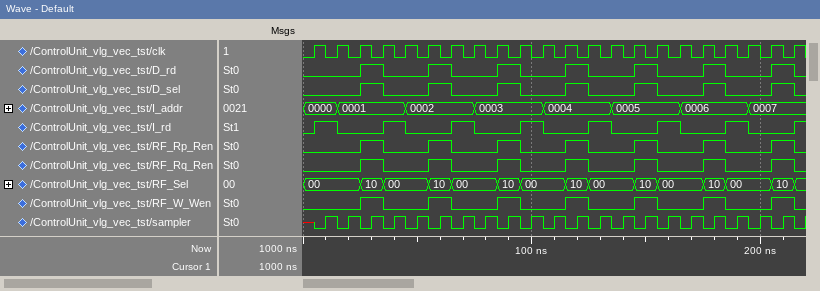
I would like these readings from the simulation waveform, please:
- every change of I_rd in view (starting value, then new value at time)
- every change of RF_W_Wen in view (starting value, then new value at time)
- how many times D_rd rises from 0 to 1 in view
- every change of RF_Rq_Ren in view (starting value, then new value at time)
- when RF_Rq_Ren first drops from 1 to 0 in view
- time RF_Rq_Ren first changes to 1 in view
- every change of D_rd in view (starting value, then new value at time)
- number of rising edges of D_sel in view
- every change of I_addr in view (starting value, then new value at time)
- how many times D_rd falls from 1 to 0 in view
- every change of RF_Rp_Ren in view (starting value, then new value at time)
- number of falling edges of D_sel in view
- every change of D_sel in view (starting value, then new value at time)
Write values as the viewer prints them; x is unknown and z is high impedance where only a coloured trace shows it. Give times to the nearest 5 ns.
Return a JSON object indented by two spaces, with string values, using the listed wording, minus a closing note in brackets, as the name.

{
  "every change of I_rd in view": "0, 1 at 5 ns, 0 at 15 ns, 1 at 35 ns, 0 at 45 ns, 1 at 65 ns, 0 at 75 ns, 1 at 95 ns, 0 at 105 ns, 1 at 125 ns, 0 at 135 ns, 1 at 155 ns, 0 at 165 ns, 1 at 185 ns, 0 at 195 ns, 1 at 215 ns",
  "every change of RF_W_Wen in view": "0, 1 at 25 ns, 0 at 35 ns, 1 at 55 ns, 0 at 65 ns, 1 at 85 ns, 0 at 95 ns, 1 at 115 ns, 0 at 125 ns, 1 at 145 ns, 0 at 155 ns, 1 at 175 ns, 0 at 185 ns, 1 at 205 ns, 0 at 215 ns",
  "how many times D_rd rises from 0 to 1 in view": "7",
  "every change of RF_Rq_Ren in view": "0, 1 at 25 ns, 0 at 35 ns, 1 at 55 ns, 0 at 65 ns, 1 at 85 ns, 0 at 95 ns, 1 at 115 ns, 0 at 125 ns, 1 at 145 ns, 0 at 155 ns, 1 at 175 ns, 0 at 185 ns, 1 at 205 ns, 0 at 215 ns",
  "when RF_Rq_Ren first drops from 1 to 0 in view": "35 ns",
  "time RF_Rq_Ren first changes to 1 in view": "25 ns",
  "every change of D_rd in view": "0, 1 at 25 ns, 0 at 35 ns, 1 at 55 ns, 0 at 65 ns, 1 at 85 ns, 0 at 95 ns, 1 at 115 ns, 0 at 125 ns, 1 at 145 ns, 0 at 155 ns, 1 at 175 ns, 0 at 185 ns, 1 at 205 ns, 0 at 215 ns",
  "number of rising edges of D_sel in view": "7",
  "every change of I_addr in view": "0000, 0001 at 15 ns, 0002 at 45 ns, 0003 at 75 ns, 0004 at 105 ns, 0005 at 135 ns, 0006 at 165 ns, 0007 at 195 ns",
  "how many times D_rd falls from 1 to 0 in view": "7",
  "every change of RF_Rp_Ren in view": "0, 1 at 25 ns, 0 at 35 ns, 1 at 55 ns, 0 at 65 ns, 1 at 85 ns, 0 at 95 ns, 1 at 115 ns, 0 at 125 ns, 1 at 145 ns, 0 at 155 ns, 1 at 175 ns, 0 at 185 ns, 1 at 205 ns, 0 at 215 ns",
  "number of falling edges of D_sel in view": "7",
  "every change of D_sel in view": "0, 1 at 25 ns, 0 at 35 ns, 1 at 55 ns, 0 at 65 ns, 1 at 85 ns, 0 at 95 ns, 1 at 115 ns, 0 at 125 ns, 1 at 145 ns, 0 at 155 ns, 1 at 175 ns, 0 at 185 ns, 1 at 205 ns, 0 at 215 ns"
}
